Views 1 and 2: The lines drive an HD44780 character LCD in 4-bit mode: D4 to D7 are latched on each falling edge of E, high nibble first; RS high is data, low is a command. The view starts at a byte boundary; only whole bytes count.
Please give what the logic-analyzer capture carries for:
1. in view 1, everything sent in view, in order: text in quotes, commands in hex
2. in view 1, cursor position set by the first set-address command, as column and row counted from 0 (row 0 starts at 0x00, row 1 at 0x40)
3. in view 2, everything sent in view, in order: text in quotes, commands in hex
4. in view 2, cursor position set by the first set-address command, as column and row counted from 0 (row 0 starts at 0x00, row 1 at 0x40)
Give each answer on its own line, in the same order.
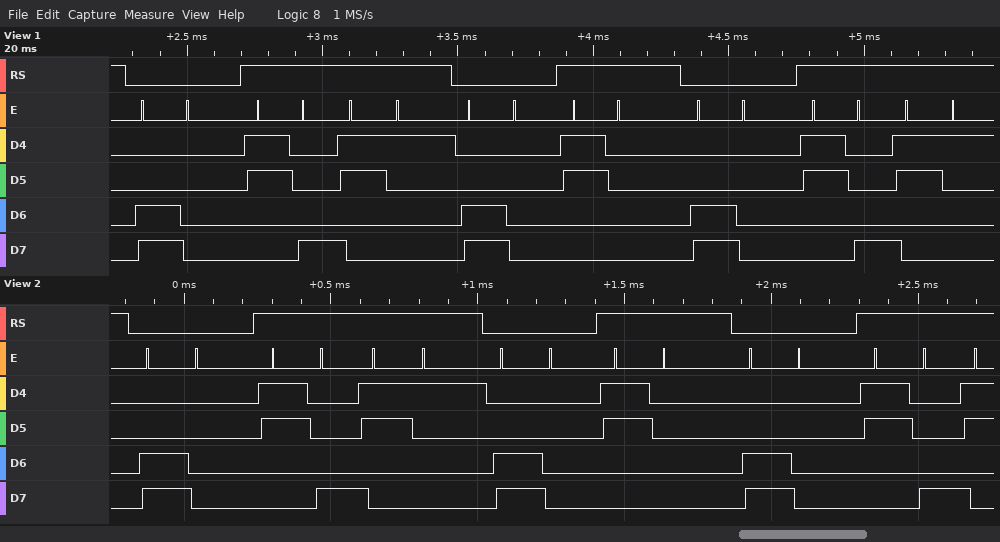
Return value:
0xC0 "81" 0xC0 "0" 0xC0 "81"
column 0, row 1
0xC0 "81" 0xC0 "0" 0xC0 "8"
column 0, row 1
